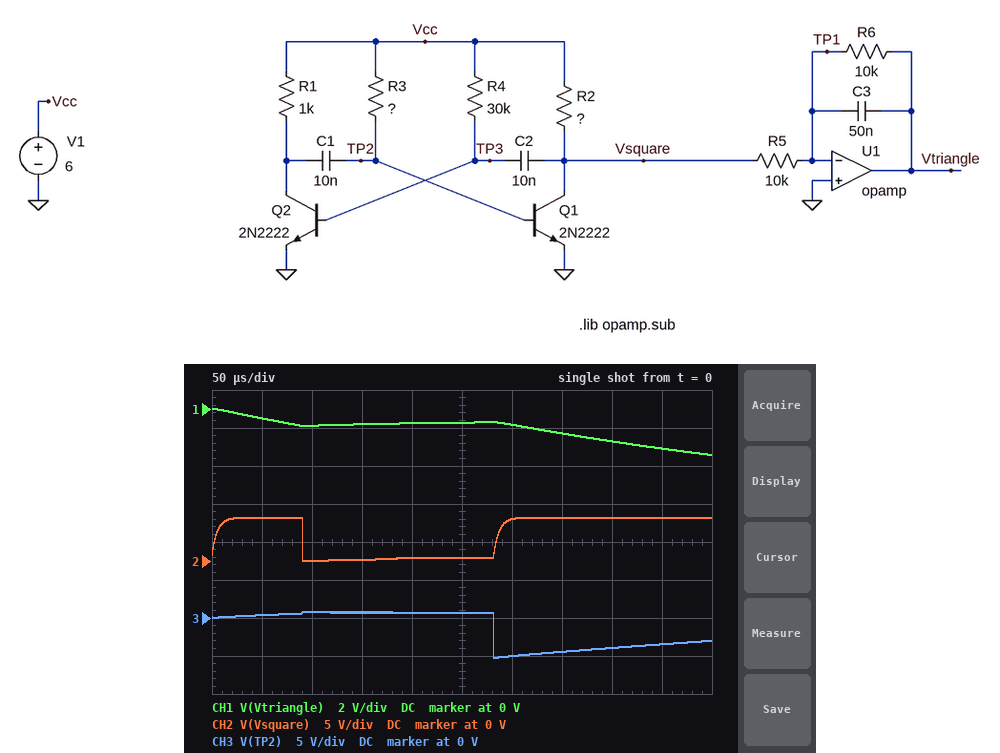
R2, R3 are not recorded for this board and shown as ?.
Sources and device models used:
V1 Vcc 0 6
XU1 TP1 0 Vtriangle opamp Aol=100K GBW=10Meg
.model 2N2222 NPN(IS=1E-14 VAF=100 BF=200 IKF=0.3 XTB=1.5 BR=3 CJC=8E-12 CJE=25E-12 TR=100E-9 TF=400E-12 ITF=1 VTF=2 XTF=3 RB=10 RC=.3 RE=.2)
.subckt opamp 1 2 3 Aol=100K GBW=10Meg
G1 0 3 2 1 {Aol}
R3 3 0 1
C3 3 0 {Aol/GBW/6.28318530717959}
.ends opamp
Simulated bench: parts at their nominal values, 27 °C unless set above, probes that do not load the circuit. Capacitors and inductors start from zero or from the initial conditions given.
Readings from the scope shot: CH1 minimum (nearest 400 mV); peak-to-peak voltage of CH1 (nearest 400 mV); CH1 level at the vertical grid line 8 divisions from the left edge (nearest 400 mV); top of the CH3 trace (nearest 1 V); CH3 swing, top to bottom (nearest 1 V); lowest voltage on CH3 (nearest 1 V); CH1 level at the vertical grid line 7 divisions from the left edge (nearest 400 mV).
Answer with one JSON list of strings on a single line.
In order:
["-2.4 V", "2.4 V", "-1.6 V", "1 V", "6 V", "-5 V", "-1.2 V"]
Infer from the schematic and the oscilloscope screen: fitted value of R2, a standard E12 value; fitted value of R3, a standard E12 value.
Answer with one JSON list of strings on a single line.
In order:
["560 Ω", "100 kΩ"]
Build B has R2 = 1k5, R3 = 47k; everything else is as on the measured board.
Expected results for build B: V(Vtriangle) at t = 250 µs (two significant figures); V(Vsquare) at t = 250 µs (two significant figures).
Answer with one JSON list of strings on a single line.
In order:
["-1.8 V", "5.2 V"]
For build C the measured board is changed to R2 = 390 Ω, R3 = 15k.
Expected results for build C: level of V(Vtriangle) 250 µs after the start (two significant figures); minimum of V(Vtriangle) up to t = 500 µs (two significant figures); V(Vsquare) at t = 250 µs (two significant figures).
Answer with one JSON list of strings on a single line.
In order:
["-360 mV", "-1.2 V", "5.8 V"]
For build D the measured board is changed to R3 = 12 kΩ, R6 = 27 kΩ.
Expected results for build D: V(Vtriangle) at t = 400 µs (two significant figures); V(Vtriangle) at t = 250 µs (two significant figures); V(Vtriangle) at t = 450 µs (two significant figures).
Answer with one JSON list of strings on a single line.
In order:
["-1.5 V", "-800 mV", "-1.6 V"]
